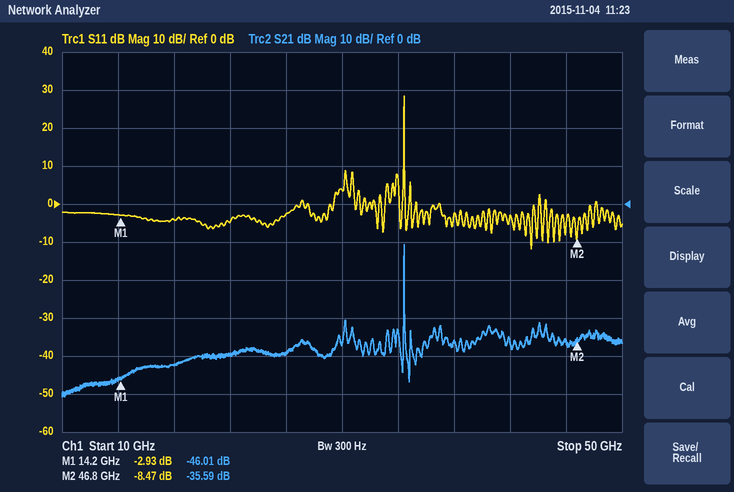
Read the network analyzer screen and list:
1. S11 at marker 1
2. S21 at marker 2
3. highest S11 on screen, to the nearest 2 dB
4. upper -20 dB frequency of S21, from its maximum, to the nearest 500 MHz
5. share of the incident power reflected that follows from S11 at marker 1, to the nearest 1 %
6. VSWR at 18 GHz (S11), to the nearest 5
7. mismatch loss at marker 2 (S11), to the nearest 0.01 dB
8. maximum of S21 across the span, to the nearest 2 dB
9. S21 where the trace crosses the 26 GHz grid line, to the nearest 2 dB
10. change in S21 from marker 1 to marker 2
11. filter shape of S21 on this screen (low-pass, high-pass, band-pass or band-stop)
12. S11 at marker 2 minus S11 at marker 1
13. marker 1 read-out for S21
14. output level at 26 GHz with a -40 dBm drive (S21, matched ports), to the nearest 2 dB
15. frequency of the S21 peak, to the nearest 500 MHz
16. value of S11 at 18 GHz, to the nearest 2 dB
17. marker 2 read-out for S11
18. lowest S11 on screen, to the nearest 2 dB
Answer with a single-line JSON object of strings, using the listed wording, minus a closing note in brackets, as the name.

{"S11 at marker 1": "-2.93 dB", "S21 at marker 2": "-35.59 dB", "highest S11 on screen, to the nearest 2 dB": "28 dB", "upper -20 dB frequency of S21, from its maximum, to the nearest 500 MHz": "34.5 GHz", "share of the incident power reflected that follows from S11 at marker 1, to the nearest 1 %": "51 %", "VSWR at 18 GHz (S11), to the nearest 5": "5", "mismatch loss at marker 2 (S11), to the nearest 0.01 dB": "0.67 dB", "maximum of S21 across the span, to the nearest 2 dB": "-10 dB", "S21 where the trace crosses the 26 GHz grid line, to the nearest 2 dB": "-40 dB", "change in S21 from marker 1 to marker 2": "10.42 dB", "filter shape of S21 on this screen": "band-pass", "S11 at marker 2 minus S11 at marker 1": "-5.54 dB", "marker 1 read-out for S21": "-46.01 dB", "output level at 26 GHz with a -40 dBm drive (S21, matched ports), to the nearest 2 dB": "-80 dBm", "frequency of the S21 peak, to the nearest 500 MHz": "34.5 GHz", "value of S11 at 18 GHz, to the nearest 2 dB": "-4 dB", "marker 2 read-out for S11": "-8.47 dB", "lowest S11 on screen, to the nearest 2 dB": "-12 dB"}
